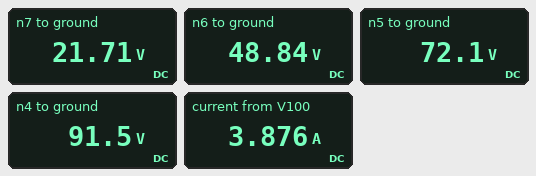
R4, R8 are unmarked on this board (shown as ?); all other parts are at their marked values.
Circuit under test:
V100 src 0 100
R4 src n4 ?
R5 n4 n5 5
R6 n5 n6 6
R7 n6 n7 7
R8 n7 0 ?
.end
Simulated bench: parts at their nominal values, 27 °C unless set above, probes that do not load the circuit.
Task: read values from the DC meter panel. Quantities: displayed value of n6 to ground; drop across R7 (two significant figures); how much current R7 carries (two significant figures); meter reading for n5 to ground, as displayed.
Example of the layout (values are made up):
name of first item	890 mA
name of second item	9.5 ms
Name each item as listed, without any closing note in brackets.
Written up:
displayed value of n6 to ground	48.84 V
drop across R7	27 V
how much current R7 carries	3.9 A
meter reading for n5 to ground, as displayed	72.1 V
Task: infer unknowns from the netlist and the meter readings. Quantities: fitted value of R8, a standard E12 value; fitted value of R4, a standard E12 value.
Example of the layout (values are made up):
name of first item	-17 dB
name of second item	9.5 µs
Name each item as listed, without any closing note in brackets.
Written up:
fitted value of R8, a standard E12 value	5.6 Ω
fitted value of R4, a standard E12 value	2.2 Ω
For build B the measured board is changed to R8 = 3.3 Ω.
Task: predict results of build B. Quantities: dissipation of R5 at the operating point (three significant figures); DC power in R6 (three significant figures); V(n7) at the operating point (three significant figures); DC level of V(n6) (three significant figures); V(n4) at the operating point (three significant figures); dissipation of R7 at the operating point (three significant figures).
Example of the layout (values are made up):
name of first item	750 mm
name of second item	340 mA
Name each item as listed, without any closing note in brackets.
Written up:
dissipation of R5 at the operating point	90.5 W
DC power in R6	109 W
V(n7) at the operating point	14.0 V
DC level of V(n6)	43.8 V
V(n4) at the operating point	90.6 V
dissipation of R7 at the operating point	127 W
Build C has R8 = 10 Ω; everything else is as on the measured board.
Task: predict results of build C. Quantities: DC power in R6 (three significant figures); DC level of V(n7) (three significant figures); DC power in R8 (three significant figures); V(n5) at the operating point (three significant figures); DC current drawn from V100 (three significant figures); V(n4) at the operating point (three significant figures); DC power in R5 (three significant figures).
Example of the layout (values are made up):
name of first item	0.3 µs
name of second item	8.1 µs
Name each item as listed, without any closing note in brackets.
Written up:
DC power in R6	65.8 W
DC level of V(n7)	33.1 V
DC power in R8	110 W
V(n5) at the operating point	76.2 V
DC current drawn from V100	3.31 A
V(n4) at the operating point	92.7 V
DC power in R5	54.8 W
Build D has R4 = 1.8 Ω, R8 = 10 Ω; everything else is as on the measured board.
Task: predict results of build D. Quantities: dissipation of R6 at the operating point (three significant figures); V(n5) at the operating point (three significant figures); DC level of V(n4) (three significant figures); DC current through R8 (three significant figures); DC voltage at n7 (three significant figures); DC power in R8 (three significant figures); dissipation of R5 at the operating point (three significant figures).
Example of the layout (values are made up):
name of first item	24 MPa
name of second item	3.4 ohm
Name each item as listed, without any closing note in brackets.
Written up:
dissipation of R6 at the operating point	67.6 W
V(n5) at the operating point	77.2 V
DC level of V(n4)	94.0 V
DC current through R8	3.36 A
DC voltage at n7	33.6 V
DC power in R8	113 W
dissipation of R5 at the operating point	56.3 W
